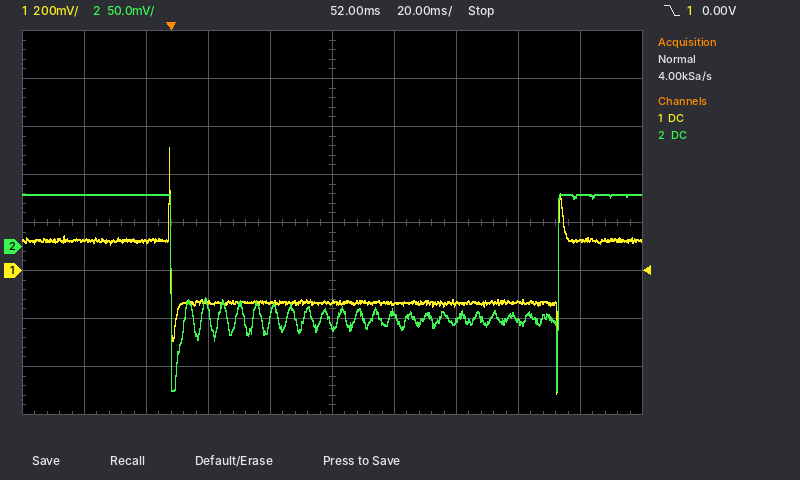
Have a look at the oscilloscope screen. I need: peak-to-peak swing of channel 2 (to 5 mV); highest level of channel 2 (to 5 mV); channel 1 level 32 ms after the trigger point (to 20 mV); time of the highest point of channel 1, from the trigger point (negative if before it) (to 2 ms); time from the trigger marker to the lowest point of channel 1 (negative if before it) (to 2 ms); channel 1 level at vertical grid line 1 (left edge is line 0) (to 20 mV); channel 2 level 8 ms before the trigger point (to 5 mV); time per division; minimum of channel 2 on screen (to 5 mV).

205 mV
55 mV
-140 mV
0 ms
+124 ms
120 mV
55 mV
20 ms
-150 mV
